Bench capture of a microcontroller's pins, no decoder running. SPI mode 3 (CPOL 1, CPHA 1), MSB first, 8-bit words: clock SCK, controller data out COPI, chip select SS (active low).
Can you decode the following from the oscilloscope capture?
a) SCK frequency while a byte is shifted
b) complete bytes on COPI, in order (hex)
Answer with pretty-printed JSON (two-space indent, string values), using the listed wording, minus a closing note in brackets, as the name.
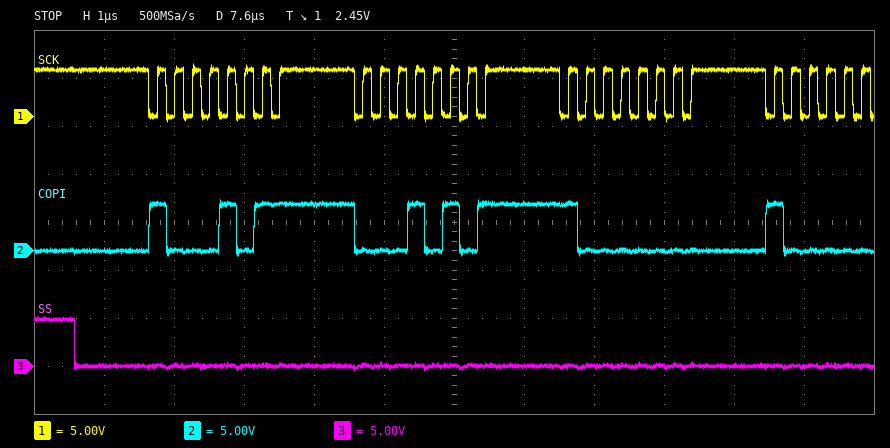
{
  "SCK frequency while a byte is shifted": "4 MHz",
  "complete bytes on COPI, in order": "8B 15 80"
}
